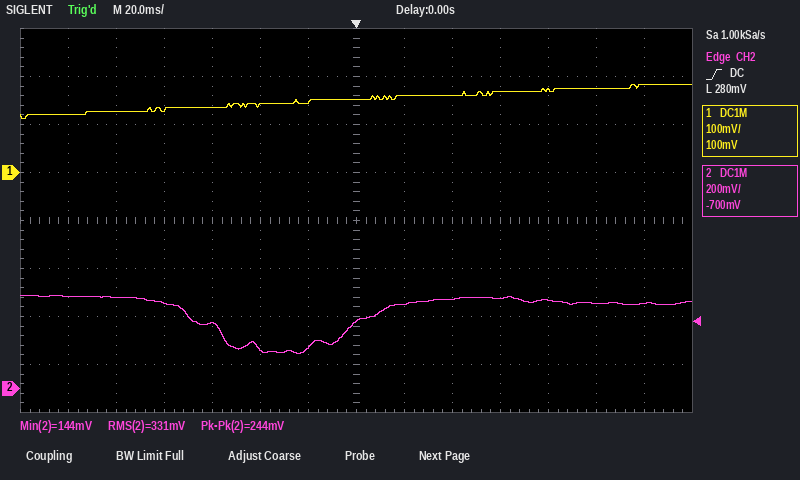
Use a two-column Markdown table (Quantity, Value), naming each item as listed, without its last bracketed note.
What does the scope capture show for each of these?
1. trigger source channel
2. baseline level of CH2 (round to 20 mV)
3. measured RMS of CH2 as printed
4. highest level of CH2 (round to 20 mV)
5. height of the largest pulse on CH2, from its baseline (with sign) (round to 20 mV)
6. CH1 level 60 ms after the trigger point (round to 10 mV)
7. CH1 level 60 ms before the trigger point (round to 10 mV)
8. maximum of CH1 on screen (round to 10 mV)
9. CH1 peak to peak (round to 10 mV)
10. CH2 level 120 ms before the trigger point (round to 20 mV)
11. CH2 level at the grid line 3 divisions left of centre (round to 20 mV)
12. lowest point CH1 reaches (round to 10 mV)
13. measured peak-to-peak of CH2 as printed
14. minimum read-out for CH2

| Quantity | Value |
|---|---|
| trigger source channel | CH2 |
| baseline level of CH2 | 360 mV |
| measured RMS of CH2 as printed | 331 mV |
| highest level of CH2 | 380 mV |
| height of the largest pulse on CH2, from its baseline (with sign) | -220 mV |
| CH1 level 60 ms after the trigger point | 170 mV |
| CH1 level 60 ms before the trigger point | 140 mV |
| maximum of CH1 on screen | 180 mV |
| CH1 peak to peak | 70 mV |
| CH2 level 120 ms before the trigger point | 380 mV |
| CH2 level at the grid line 3 divisions left of centre | 280 mV |
| lowest point CH1 reaches | 110 mV |
| measured peak-to-peak of CH2 as printed | 244 mV |
| minimum read-out for CH2 | 144 mV |
